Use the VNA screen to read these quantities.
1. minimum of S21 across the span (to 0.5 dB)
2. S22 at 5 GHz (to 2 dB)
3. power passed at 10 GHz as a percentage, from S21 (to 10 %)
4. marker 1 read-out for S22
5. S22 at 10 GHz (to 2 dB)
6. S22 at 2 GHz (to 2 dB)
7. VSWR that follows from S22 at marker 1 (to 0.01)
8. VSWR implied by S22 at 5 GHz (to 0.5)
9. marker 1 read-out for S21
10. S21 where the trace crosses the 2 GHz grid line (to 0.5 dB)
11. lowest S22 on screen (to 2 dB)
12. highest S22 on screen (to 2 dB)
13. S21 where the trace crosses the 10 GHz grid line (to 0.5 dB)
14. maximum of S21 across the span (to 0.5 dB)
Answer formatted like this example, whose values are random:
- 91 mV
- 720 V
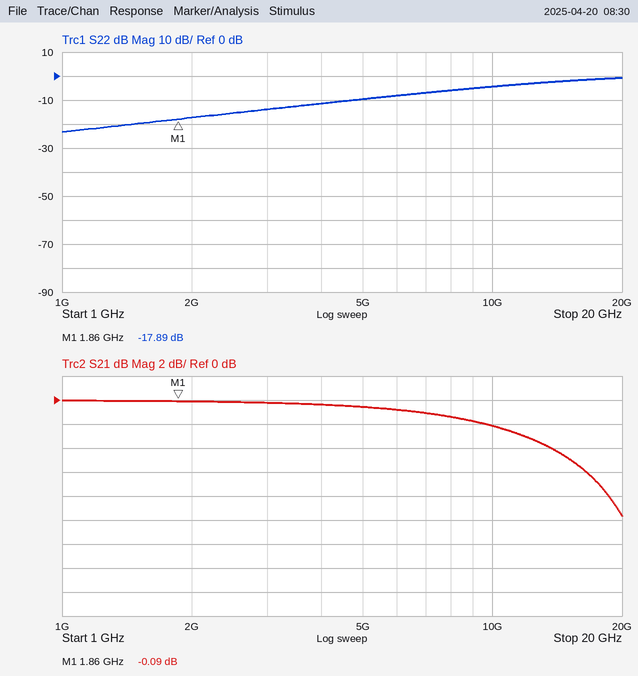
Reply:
- -9.5 dB
- -10 dB
- 60 %
- -17.89 dB
- -4 dB
- -18 dB
- 1.29
- 2.0
- -0.09 dB
- 0.0 dB
- -24 dB
- 0 dB
- -2.0 dB
- 0.0 dB
